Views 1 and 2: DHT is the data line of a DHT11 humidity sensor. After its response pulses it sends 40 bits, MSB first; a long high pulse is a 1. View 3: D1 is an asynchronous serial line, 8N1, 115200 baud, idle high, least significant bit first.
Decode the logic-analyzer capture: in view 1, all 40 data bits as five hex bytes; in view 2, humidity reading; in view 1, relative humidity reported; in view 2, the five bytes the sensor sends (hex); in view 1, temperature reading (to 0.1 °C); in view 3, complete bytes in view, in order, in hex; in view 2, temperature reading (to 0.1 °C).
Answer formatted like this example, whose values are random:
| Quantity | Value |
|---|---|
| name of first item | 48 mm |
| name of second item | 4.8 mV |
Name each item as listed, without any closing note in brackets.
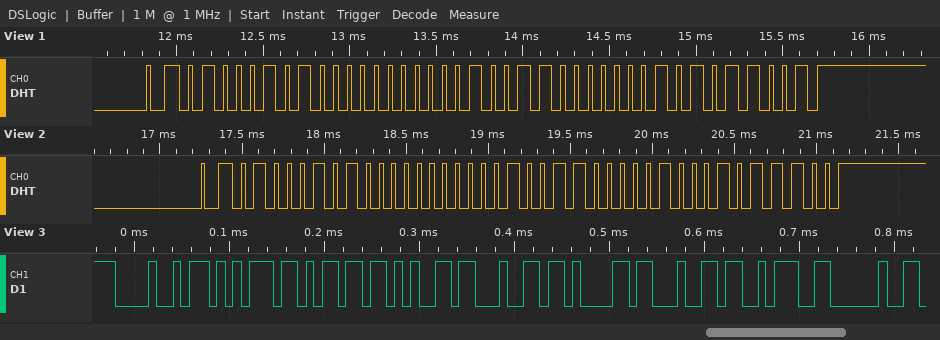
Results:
| Quantity | Value |
|---|---|
| in view 1, all 40 data bits as five hex bytes | 45 00 13 01 59 |
| in view 2, humidity reading | 69 % |
| in view 1, relative humidity reported | 69 % |
| in view 2, the five bytes the sensor sends | 45 00 13 04 5C |
| in view 1, temperature reading | 19.1 °C |
| in view 3, complete bytes in view, in order, in hex | 48 75 6D 65 64 61 64 3A 20 |
| in view 2, temperature reading | 19.4 °C |
